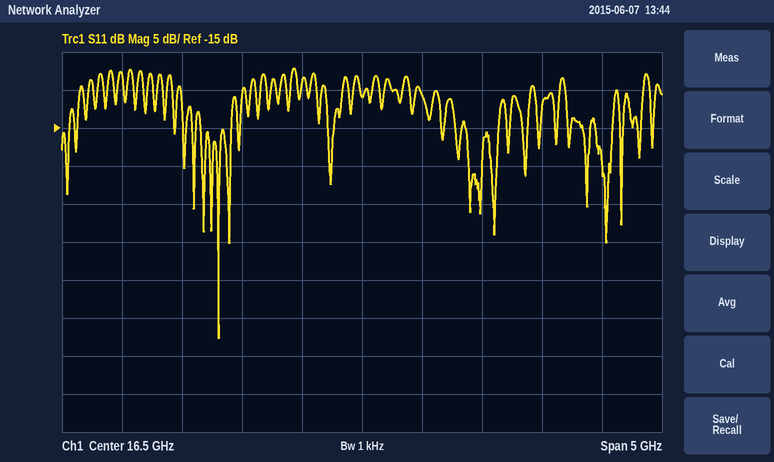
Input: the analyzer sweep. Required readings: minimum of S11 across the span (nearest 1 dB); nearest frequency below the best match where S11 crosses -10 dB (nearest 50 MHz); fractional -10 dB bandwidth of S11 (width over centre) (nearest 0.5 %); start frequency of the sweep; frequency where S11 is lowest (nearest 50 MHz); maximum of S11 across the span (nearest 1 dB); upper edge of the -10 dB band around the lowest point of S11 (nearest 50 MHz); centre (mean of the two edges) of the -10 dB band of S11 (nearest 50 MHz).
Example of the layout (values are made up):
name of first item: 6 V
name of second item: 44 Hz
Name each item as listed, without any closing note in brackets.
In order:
minimum of S11 across the span: -43 dB
nearest frequency below the best match where S11 crosses -10 dB: 15.00 GHz
fractional -10 dB bandwidth of S11 (width over centre): 3.5 %
start frequency of the sweep: 14 GHz
frequency where S11 is lowest: 15.30 GHz
maximum of S11 across the span: -7 dB
upper edge of the -10 dB band around the lowest point of S11: 15.50 GHz
centre (mean of the two edges) of the -10 dB band of S11: 15.25 GHz
